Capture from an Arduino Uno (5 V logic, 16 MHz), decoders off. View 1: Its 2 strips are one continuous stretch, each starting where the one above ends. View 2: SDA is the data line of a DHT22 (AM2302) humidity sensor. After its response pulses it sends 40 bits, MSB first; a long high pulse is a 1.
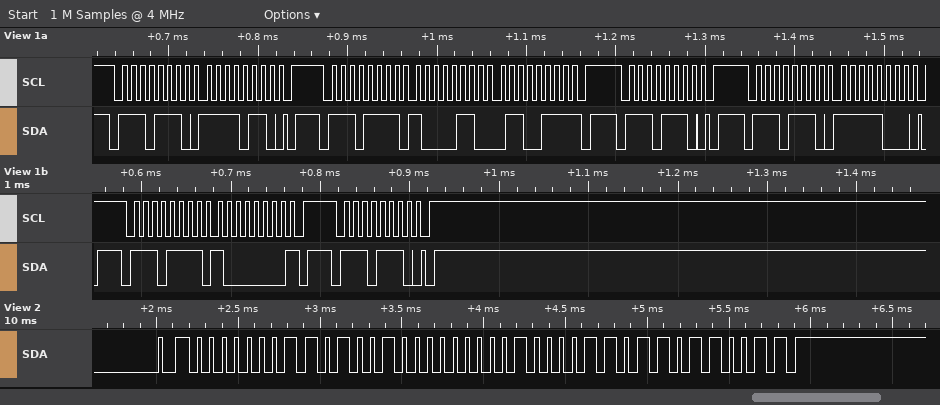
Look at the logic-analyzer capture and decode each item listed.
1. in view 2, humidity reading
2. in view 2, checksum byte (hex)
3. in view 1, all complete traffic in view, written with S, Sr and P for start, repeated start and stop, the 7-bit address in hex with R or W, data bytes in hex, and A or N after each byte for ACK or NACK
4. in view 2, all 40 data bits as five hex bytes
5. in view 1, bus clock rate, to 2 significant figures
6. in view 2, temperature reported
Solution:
42.0 %
0xB3
S 77W A F6 A P S 77R A 86 A 67 N P S 77W A P S 77W A F8 A P S 77R A 80 N P S 77W A P
01 A4 01 0D B3
100 kHz
26.9 °C
